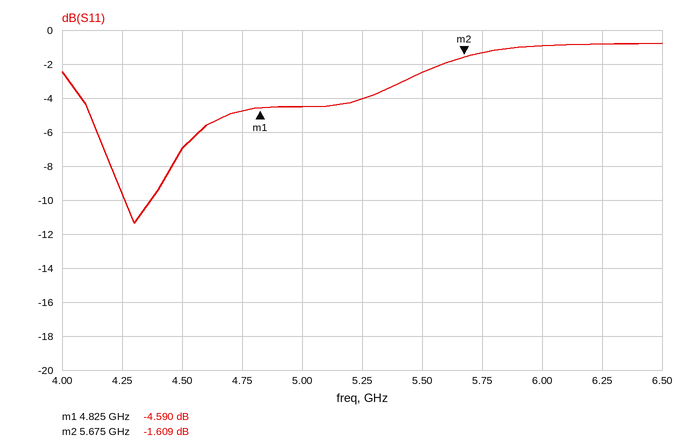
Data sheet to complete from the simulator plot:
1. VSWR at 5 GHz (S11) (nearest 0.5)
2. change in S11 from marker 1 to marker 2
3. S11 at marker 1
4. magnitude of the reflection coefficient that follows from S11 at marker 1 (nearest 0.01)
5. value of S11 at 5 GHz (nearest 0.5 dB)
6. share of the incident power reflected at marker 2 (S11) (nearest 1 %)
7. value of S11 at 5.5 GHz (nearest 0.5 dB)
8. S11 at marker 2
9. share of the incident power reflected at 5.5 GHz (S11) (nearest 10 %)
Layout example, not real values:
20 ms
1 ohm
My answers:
4.0
2.981 dB
-4.590 dB
0.59
-4.5 dB
69 %
-2.5 dB
-1.609 dB
60 %
